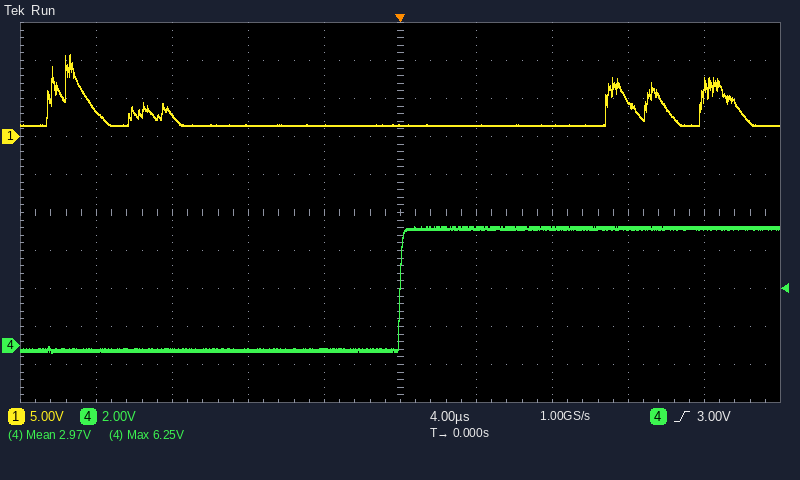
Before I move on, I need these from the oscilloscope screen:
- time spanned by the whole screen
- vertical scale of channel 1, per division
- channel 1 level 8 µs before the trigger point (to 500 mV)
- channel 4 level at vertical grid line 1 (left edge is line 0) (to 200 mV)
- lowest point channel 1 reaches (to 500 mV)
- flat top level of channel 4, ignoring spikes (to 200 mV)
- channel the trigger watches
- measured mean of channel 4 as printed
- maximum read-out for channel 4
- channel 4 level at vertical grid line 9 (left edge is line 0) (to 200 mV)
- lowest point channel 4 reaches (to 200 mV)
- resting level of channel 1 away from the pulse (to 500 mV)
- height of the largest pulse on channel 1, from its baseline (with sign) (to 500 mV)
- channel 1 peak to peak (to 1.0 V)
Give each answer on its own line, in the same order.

40 µs
5 V
1.5 V
-200 mV
1.5 V
6.2 V
channel 4
2.97 V
6.25 V
6.2 V
-400 mV
1.5 V
+9.5 V
9.0 V
